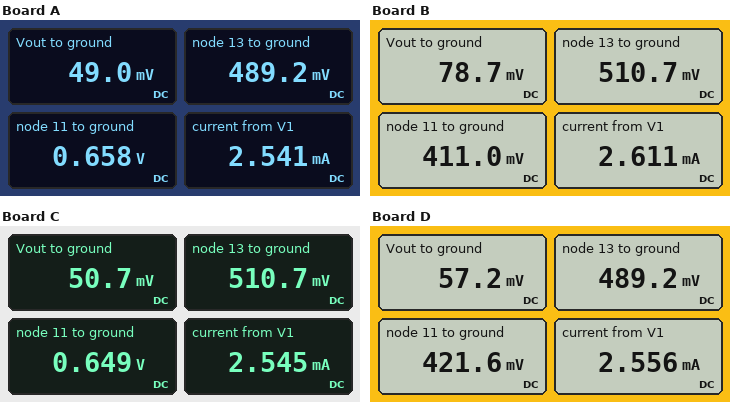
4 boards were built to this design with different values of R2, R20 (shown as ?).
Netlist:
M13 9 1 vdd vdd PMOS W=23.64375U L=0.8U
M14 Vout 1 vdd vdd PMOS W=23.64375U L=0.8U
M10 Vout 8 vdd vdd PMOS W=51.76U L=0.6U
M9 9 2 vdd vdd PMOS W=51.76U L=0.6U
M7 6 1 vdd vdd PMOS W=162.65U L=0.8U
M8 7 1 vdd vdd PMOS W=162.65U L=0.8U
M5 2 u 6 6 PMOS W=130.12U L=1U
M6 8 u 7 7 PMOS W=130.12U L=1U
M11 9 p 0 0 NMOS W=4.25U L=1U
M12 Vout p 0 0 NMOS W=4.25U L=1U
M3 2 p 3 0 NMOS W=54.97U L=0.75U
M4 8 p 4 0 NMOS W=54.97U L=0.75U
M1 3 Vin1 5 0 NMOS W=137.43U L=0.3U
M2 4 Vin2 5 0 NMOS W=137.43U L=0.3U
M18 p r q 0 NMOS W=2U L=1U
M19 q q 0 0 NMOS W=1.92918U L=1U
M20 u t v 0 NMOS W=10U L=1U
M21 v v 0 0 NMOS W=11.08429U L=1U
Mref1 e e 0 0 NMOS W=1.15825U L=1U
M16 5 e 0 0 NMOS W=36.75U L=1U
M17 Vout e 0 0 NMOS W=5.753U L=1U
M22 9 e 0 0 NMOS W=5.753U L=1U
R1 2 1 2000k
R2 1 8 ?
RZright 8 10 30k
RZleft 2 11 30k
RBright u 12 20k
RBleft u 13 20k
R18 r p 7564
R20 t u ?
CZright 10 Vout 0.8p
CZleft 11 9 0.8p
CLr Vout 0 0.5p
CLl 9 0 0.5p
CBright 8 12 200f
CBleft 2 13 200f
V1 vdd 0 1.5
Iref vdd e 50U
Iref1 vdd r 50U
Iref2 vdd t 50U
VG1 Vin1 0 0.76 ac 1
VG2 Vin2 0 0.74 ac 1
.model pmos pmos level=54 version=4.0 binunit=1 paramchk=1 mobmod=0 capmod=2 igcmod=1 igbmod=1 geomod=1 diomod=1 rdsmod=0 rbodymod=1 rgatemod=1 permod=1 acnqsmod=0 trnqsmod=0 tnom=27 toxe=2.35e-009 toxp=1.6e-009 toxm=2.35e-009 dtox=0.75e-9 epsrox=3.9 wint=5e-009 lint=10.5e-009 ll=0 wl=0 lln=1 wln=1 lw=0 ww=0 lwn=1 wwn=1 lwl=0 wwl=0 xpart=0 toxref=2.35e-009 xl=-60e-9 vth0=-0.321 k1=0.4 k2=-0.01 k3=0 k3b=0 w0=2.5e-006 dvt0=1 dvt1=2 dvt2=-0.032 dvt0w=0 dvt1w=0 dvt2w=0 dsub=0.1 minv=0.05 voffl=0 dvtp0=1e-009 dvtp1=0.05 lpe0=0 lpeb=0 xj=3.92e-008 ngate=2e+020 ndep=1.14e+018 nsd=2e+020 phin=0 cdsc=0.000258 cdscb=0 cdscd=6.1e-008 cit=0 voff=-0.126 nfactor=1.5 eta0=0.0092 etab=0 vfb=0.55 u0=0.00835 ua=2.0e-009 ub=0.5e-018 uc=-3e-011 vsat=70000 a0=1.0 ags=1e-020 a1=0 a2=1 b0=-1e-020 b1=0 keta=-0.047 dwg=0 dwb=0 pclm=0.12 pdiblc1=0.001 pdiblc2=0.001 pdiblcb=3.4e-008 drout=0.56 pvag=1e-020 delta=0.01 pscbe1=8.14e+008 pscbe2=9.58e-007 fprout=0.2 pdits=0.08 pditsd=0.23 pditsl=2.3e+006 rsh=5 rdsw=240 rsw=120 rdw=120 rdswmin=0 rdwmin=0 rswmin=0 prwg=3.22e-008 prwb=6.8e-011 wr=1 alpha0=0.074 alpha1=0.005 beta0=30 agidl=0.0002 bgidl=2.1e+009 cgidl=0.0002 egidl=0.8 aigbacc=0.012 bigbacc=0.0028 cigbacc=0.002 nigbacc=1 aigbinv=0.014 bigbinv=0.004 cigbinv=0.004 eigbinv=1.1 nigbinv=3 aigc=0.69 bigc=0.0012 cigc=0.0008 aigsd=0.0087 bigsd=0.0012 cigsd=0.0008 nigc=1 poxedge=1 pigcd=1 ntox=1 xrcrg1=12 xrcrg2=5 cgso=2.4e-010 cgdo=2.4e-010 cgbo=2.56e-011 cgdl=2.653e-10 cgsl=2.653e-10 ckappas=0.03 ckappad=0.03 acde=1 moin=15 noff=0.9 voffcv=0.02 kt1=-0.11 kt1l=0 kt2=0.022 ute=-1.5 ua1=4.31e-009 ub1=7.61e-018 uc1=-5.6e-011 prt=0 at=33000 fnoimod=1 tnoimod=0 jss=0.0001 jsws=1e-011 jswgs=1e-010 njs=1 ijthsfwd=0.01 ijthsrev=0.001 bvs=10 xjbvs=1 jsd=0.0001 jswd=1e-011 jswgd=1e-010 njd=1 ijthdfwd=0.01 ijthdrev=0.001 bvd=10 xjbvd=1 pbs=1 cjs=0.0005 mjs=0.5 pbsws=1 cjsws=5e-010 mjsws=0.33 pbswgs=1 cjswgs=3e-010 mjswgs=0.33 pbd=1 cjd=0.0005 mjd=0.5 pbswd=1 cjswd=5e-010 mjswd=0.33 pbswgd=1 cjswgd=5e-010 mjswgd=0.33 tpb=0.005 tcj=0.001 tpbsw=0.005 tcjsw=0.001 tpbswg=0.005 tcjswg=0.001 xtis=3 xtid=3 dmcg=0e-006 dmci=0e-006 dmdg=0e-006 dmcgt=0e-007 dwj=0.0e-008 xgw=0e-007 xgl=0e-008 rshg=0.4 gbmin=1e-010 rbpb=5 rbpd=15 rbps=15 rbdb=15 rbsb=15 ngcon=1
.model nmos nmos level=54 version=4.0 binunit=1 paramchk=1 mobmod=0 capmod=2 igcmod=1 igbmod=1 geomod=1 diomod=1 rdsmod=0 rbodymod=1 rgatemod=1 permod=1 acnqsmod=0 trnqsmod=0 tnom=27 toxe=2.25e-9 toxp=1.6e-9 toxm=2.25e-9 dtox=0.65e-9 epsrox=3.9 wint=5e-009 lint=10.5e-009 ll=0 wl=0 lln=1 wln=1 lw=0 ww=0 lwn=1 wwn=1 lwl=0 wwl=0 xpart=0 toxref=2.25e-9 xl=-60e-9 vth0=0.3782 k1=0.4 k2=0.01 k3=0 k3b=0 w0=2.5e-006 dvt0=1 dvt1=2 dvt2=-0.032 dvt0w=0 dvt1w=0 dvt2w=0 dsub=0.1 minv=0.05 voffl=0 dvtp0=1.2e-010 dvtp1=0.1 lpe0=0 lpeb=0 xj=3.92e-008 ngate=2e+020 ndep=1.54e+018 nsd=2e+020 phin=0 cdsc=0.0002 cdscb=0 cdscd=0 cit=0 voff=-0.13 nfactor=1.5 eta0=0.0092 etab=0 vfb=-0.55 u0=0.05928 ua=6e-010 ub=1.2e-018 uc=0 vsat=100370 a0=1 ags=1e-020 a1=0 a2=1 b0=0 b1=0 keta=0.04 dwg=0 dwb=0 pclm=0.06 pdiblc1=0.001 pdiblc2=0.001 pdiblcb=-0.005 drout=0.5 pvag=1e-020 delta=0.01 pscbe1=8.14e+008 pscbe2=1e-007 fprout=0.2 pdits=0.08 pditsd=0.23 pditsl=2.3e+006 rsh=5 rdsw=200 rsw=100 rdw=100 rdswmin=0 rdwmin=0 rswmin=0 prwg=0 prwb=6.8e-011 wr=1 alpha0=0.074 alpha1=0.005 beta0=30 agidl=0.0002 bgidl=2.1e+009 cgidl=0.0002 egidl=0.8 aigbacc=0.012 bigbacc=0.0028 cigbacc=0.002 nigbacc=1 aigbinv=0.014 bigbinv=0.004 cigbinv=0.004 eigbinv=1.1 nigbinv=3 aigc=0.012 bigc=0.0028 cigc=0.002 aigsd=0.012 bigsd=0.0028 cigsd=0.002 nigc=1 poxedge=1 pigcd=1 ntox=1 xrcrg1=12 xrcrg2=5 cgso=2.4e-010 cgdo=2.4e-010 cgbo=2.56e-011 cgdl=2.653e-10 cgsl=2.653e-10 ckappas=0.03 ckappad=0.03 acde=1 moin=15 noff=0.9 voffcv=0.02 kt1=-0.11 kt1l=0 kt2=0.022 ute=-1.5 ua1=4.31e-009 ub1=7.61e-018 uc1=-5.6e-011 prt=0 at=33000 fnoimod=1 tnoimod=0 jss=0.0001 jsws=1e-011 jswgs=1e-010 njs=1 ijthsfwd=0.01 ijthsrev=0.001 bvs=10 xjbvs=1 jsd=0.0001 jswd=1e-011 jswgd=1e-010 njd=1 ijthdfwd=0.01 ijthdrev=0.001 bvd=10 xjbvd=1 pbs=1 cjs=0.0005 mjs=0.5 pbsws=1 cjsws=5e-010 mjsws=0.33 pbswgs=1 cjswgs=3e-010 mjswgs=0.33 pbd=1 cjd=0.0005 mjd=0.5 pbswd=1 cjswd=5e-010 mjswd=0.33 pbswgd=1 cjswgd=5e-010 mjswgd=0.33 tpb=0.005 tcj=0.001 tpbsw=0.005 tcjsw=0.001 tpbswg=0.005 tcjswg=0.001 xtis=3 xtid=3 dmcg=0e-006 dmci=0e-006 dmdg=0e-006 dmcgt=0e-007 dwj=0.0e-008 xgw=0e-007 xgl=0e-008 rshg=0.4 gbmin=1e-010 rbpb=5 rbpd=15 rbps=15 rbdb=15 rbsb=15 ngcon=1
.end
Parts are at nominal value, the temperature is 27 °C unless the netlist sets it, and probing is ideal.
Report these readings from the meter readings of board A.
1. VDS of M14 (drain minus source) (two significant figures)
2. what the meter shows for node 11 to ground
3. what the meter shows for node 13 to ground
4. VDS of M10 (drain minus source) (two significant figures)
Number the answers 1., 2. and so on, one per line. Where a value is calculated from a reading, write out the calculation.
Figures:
1. 49 mV - 1.5 V = -1.5 V
2. 0.658 V
3. 489.2 mV
4. 49 mV - 1.5 V = -1.5 V
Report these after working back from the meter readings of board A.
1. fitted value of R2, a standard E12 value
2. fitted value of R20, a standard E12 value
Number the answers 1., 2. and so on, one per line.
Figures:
1. 3.9 MΩ
2. 15 kΩ
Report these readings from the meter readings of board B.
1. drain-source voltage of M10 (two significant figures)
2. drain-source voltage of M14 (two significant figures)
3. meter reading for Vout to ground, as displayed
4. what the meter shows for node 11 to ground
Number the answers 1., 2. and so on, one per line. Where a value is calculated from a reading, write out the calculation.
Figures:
1. 78.7 mV - 1.5 V = -1.4 V
2. 78.7 mV - 1.5 V = -1.4 V
3. 78.7 mV
4. 411.0 mV
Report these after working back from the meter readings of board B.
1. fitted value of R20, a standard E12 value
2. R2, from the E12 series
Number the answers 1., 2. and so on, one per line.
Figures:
1. 12 kΩ
2. 680 kΩ
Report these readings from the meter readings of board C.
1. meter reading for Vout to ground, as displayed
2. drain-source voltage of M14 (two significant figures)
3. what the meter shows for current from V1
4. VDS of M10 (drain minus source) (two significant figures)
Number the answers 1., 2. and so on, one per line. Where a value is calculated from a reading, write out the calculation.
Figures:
1. 50.7 mV
2. 50.7 mV - 1.5 V = -1.4 V
3. 2.545 mA
4. 50.7 mV - 1.5 V = -1.4 V
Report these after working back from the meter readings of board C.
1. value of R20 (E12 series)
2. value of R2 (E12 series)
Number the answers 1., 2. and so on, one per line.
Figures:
1. 12 kΩ
2. 3.9 MΩ
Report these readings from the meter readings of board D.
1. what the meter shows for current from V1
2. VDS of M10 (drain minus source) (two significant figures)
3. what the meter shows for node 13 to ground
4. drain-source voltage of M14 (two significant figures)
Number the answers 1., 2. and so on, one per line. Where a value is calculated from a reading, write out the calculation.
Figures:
1. 2.556 mA
2. 57.2 mV - 1.5 V = -1.4 V
3. 489.2 mV
4. 57.2 mV - 1.5 V = -1.4 V
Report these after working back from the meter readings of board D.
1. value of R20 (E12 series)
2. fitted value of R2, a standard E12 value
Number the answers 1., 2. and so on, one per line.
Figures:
1. 15 kΩ
2. 1 MΩ
